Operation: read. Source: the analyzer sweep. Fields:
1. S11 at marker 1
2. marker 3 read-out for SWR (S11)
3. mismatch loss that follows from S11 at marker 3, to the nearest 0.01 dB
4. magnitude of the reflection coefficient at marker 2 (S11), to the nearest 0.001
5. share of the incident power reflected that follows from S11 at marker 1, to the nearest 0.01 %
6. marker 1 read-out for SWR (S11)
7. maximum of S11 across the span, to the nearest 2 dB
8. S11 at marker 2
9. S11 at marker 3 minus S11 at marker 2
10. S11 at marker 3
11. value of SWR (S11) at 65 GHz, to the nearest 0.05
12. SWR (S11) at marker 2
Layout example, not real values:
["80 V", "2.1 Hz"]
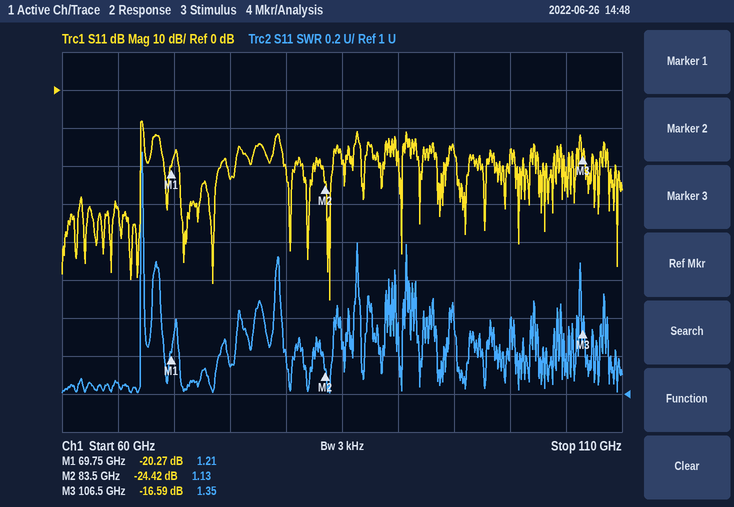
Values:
["-20.27 dB", "1.35", "0.10 dB", "0.060", "0.94 %", "1.21", "-8 dB", "-24.42 dB", "7.83 dB", "-16.59 dB", "1.05", "1.13"]
